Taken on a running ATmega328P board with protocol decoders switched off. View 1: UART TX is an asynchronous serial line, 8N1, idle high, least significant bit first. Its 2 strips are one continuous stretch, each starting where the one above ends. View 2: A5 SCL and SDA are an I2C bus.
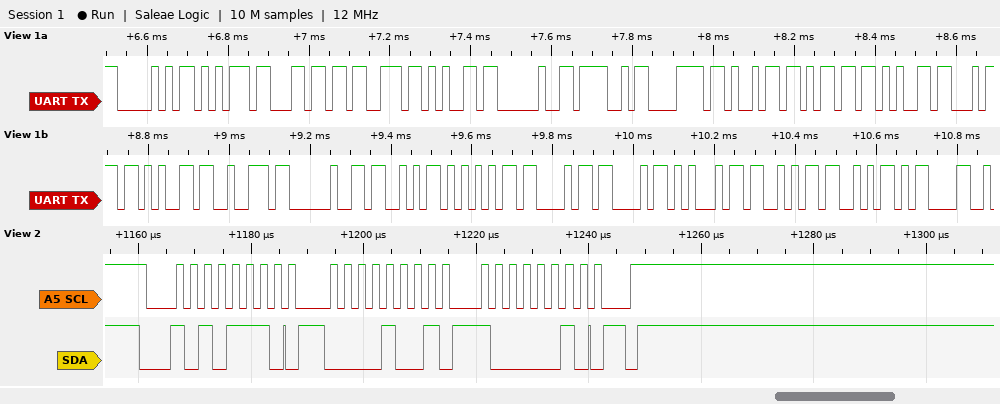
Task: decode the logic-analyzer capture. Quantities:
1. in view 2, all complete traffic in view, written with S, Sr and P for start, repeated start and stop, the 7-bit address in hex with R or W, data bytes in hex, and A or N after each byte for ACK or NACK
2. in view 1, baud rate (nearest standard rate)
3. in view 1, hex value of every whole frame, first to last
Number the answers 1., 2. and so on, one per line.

1. S 57W A 09 A 82 A P
2. 57600 baud
3. 50 75 6C 73 65 20 4F 78 69 6D 65 74 65 72 20 53 55 43 43 45 53 53 0D
